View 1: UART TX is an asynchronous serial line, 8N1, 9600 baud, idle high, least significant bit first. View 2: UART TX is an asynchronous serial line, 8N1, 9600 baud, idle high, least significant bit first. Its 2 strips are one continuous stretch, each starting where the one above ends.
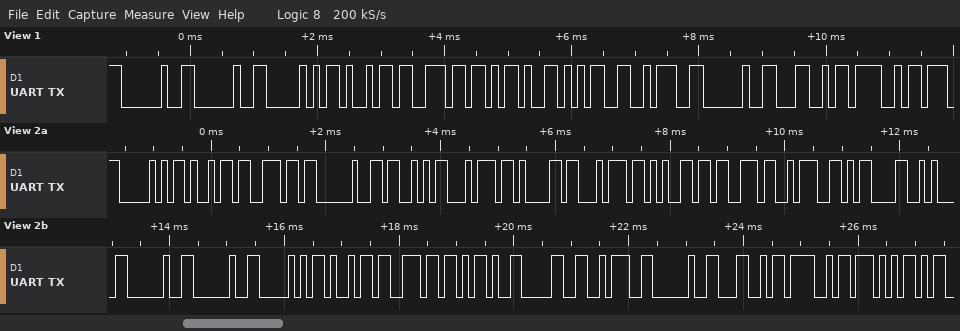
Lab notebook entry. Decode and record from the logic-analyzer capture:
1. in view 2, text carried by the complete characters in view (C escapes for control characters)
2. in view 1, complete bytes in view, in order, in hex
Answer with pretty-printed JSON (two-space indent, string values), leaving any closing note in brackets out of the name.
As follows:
{
  "in view 2, text carried by the complete characters in view": "\"Pin States:\\r\\n  Pin-0: LOW\"",
  "in view 1, complete bytes in view, in order, in hex": "0x20 0x20 0x50 0x69 0x6E 0x2D 0x35 0x3A 0x20 0x4C 0x4F"
}
